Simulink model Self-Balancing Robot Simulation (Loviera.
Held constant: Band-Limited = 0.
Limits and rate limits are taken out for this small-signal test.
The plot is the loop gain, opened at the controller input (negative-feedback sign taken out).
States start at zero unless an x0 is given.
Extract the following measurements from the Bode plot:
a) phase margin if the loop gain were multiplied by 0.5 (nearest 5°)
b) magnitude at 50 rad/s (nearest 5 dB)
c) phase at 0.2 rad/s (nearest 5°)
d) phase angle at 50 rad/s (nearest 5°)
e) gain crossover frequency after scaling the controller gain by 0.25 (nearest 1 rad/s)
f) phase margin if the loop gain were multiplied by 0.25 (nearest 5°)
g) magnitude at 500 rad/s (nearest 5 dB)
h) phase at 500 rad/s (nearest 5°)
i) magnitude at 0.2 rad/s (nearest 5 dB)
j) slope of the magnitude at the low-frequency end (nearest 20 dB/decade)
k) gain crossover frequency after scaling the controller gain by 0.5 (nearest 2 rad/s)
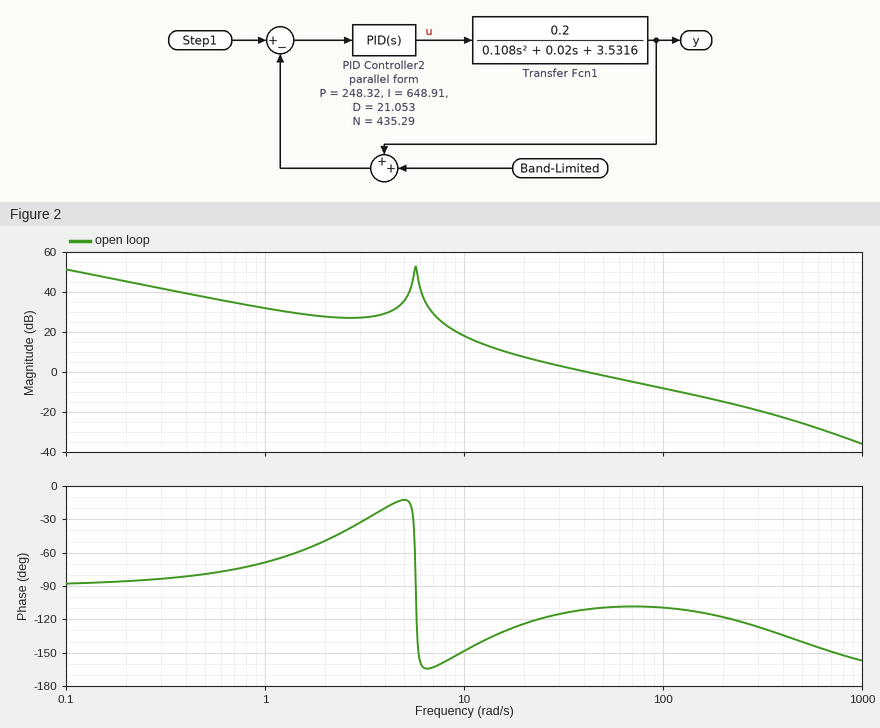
60°
0 dB
-85°
-110°
14 rad/s
45°
-25 dB
-140°
45 dB
-20 dB/decade
22 rad/s
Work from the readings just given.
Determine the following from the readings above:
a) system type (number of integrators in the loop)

1
